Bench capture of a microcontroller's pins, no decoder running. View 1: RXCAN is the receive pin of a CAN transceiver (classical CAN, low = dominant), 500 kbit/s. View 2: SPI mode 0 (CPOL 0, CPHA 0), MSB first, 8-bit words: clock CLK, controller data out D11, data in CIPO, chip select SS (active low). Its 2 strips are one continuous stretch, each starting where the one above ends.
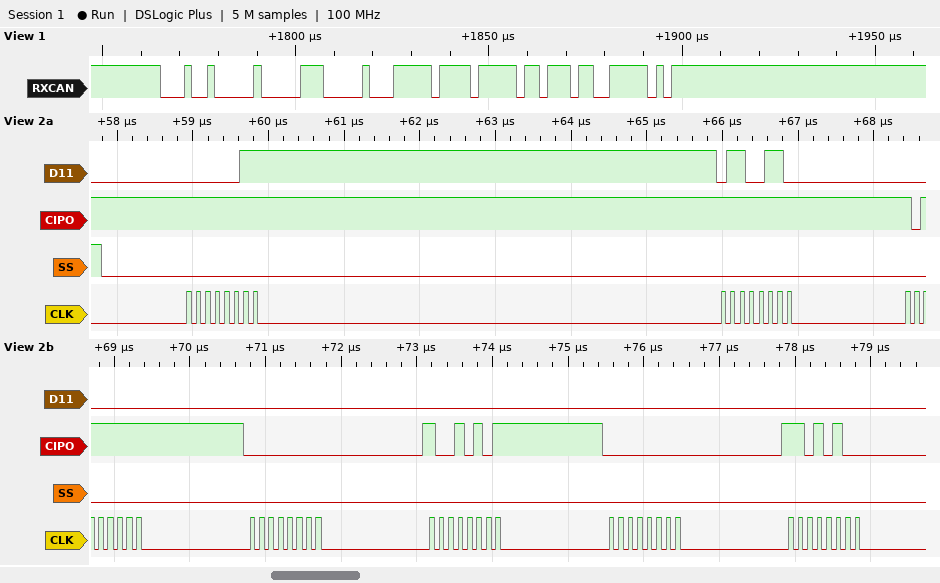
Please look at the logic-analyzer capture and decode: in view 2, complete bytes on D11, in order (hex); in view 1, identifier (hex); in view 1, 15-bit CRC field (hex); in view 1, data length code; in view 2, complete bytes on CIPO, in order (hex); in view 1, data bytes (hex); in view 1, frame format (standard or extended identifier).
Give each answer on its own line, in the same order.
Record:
0x03 0x66 0x00 0x00 0x00 0x00 0x00
0x120
0x5D9F
3
0xFF 0xFF 0xBF 0x00 0x95 0x00 0xD4
00 FF BF
standard
